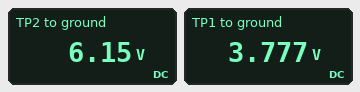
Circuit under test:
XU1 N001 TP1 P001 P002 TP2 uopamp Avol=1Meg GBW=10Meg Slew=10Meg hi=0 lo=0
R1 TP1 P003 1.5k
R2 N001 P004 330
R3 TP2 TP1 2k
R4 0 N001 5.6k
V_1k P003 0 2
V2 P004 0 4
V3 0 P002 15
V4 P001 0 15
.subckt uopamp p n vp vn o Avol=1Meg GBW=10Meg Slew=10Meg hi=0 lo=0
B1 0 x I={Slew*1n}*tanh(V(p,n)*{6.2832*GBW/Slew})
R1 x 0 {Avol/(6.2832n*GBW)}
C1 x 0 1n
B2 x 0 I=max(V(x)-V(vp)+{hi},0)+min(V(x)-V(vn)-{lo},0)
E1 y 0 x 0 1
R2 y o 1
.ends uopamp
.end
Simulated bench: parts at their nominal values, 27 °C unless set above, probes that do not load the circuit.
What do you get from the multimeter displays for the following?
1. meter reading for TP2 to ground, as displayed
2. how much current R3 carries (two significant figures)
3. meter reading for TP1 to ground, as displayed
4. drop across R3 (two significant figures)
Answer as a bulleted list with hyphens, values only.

- 6.15 V
- 1.2 mA
- 3.777 V
- 2.4 V
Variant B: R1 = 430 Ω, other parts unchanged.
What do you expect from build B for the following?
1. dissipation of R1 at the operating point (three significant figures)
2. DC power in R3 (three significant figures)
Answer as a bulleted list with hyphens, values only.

- 7.35 mW
- 34.2 mW
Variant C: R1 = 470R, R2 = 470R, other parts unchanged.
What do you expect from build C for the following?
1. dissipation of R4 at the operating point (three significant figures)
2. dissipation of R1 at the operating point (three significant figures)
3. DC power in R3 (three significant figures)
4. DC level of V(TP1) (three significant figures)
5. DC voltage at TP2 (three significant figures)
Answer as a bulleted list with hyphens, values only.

- 2.43 mW
- 6.08 mW
- 25.9 mW
- 3.69 V
- 10.9 V
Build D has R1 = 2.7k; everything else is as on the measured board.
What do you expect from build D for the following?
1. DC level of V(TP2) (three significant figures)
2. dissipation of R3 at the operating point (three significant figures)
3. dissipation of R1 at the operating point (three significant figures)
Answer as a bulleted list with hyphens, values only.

- 5.09 V
- 867 µW
- 1.17 mW
